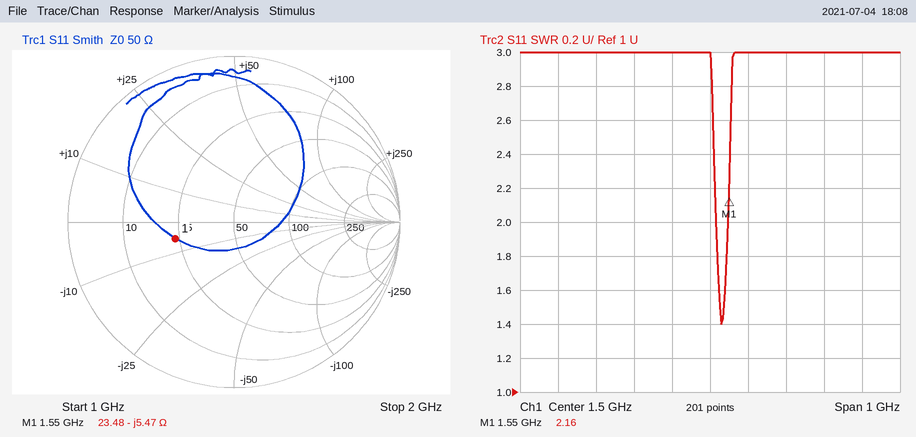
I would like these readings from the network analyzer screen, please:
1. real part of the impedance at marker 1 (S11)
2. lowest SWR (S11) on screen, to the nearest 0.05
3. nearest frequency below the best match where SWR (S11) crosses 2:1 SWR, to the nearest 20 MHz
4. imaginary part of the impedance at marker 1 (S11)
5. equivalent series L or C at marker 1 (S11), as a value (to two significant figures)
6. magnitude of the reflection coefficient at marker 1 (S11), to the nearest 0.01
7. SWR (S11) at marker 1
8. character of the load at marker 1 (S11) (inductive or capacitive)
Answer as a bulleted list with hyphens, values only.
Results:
- 23.48 Ω
- 1.40
- 1.52 GHz
- -5.47 Ω
- 19 pF
- 0.37
- 2.16
- capacitive
